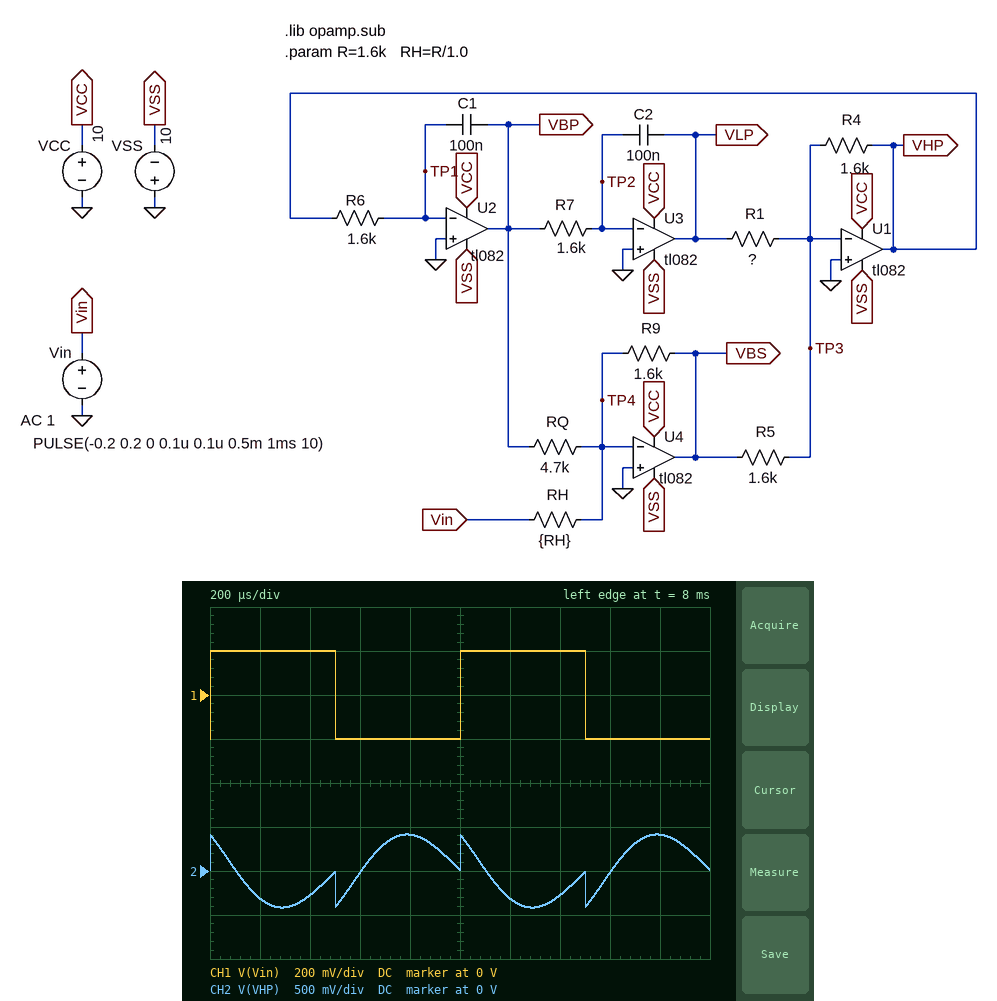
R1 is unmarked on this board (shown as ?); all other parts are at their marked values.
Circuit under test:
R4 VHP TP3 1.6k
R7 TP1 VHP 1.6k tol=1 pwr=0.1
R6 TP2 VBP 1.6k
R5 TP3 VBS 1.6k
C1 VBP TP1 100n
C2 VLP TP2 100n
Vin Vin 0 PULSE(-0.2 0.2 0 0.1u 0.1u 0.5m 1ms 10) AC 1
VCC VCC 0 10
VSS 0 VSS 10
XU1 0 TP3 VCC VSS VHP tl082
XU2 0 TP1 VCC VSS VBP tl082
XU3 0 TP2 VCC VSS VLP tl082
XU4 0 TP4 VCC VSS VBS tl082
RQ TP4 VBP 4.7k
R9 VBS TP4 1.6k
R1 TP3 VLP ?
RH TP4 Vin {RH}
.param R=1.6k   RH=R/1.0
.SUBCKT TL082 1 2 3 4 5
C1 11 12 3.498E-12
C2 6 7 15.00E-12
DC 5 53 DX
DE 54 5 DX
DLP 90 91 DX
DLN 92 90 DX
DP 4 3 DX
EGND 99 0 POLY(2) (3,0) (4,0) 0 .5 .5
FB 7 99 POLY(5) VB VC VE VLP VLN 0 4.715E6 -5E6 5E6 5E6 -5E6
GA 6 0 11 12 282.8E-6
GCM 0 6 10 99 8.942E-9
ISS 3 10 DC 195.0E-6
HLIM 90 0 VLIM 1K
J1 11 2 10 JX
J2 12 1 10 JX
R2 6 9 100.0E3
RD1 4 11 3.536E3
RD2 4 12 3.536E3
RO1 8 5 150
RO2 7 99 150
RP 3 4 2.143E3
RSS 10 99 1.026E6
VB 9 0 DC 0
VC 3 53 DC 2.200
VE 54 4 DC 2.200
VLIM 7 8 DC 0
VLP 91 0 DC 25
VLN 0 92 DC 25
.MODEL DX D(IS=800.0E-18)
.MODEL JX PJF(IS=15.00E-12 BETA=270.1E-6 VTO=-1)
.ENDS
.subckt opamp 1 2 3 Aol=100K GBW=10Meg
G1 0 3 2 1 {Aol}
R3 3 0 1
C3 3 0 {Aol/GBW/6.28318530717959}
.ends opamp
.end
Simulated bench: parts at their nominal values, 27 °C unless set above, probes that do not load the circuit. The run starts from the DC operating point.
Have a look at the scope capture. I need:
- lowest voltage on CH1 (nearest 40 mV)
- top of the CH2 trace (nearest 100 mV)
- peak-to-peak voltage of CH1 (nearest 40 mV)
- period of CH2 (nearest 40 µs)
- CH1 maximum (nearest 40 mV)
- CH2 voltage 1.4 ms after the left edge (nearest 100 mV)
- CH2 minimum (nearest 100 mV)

-200 mV
400 mV
400 mV
1.00 ms
200 mV
-300 mV
-400 mV
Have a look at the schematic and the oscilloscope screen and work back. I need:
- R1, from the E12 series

1 kΩ
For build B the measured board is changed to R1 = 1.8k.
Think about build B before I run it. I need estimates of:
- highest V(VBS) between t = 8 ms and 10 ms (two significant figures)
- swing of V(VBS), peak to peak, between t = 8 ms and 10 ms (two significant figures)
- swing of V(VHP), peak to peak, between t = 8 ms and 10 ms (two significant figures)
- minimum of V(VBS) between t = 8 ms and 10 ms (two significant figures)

300 mV
600 mV
1.8 V
-300 mV
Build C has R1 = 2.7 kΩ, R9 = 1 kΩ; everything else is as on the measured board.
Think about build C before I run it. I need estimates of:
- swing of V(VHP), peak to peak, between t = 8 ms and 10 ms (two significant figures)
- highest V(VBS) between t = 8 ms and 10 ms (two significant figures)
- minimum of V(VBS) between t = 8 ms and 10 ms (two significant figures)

680 mV
200 mV
-200 mV
